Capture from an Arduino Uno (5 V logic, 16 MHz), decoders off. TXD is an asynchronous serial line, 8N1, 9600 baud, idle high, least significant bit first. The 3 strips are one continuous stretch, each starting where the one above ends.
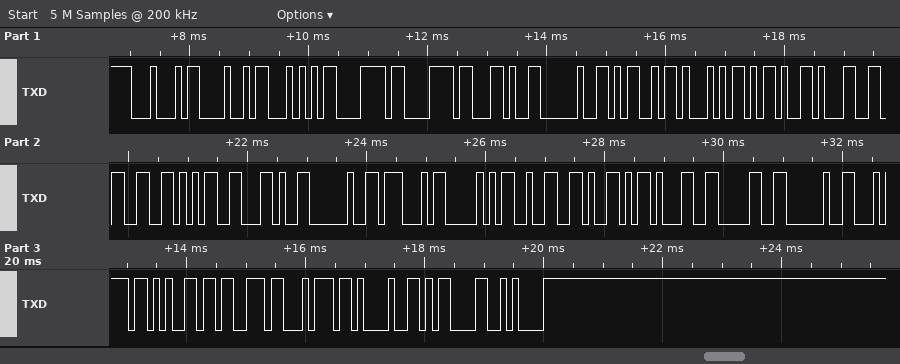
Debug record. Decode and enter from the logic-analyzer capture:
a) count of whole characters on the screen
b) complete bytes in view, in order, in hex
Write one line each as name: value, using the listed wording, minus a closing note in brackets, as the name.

count of whole characters on the screen: 29
complete bytes in view, in order, in hex: 44 48 54 78 78 2C 20 4D 51 2D 31 33 35 2C 20 47 50 32 59 31 30 20 74 65 73 74 21 0D 0A
